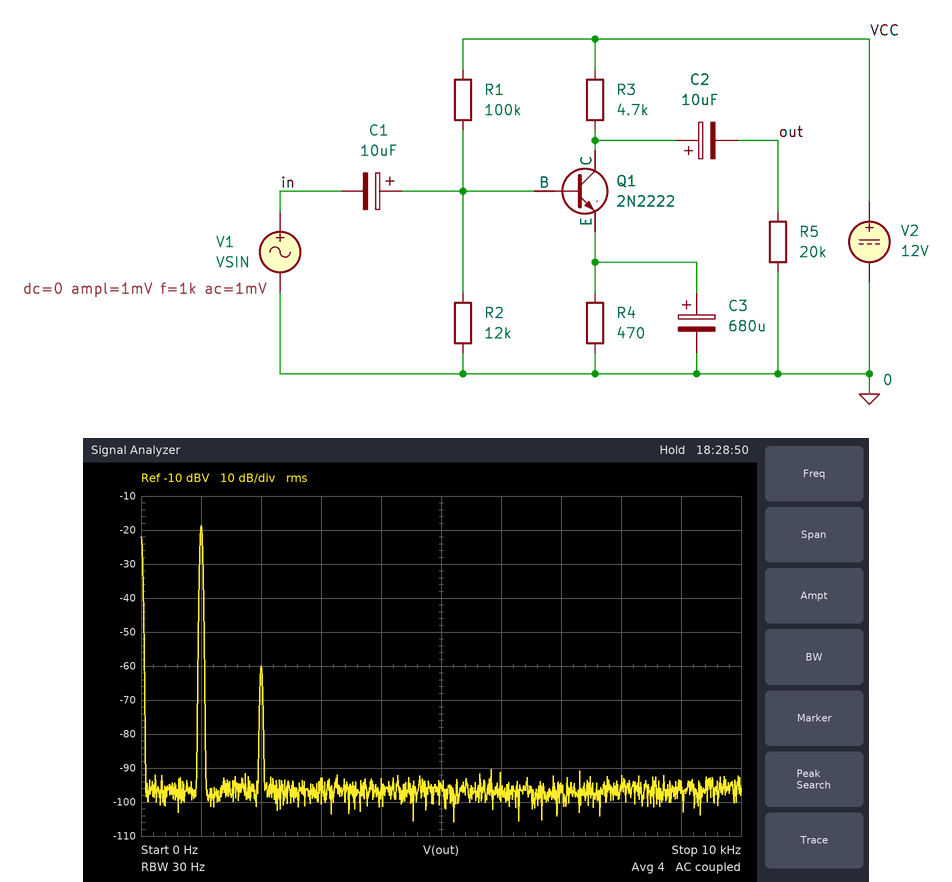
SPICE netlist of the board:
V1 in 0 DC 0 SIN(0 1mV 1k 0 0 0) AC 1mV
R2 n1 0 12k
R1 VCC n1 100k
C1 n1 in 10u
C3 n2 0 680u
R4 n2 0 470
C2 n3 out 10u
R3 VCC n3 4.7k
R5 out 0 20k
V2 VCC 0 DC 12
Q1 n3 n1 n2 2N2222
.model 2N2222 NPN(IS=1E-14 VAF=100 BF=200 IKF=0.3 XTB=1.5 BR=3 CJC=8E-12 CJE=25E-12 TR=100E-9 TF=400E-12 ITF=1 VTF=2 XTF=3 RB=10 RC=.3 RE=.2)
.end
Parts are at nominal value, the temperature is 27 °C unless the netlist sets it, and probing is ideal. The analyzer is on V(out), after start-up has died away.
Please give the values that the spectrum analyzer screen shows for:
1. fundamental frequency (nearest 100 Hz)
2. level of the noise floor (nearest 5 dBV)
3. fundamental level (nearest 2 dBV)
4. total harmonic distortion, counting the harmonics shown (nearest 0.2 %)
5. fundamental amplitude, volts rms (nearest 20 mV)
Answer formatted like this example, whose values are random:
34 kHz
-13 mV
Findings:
1.0 kHz
-95 dBV
-18 dBV
0.8 %
120 mV
